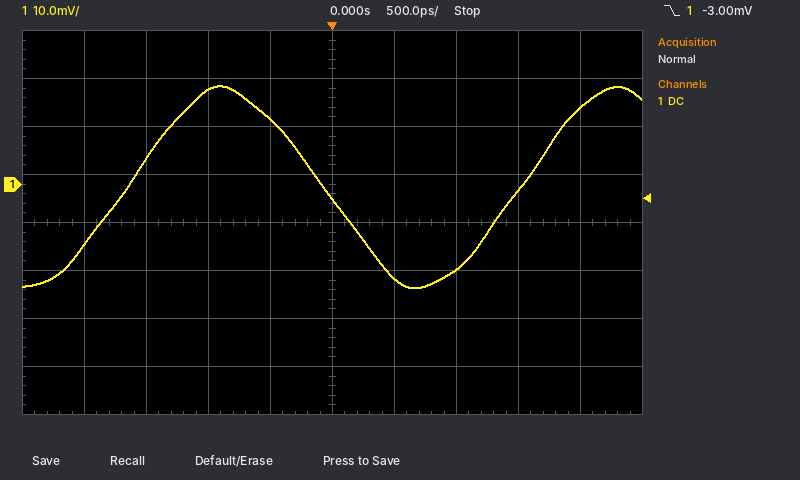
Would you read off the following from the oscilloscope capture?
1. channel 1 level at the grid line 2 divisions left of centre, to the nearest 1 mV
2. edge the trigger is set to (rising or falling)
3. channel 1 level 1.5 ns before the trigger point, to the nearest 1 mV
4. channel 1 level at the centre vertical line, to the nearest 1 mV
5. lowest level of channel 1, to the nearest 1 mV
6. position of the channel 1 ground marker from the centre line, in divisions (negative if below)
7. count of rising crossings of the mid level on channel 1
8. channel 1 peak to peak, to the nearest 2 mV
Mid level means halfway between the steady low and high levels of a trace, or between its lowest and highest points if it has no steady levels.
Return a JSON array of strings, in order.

["20 mV", "falling", "5 mV", "-3 mV", "-22 mV", "+0.8 div", "2", "42 mV"]
